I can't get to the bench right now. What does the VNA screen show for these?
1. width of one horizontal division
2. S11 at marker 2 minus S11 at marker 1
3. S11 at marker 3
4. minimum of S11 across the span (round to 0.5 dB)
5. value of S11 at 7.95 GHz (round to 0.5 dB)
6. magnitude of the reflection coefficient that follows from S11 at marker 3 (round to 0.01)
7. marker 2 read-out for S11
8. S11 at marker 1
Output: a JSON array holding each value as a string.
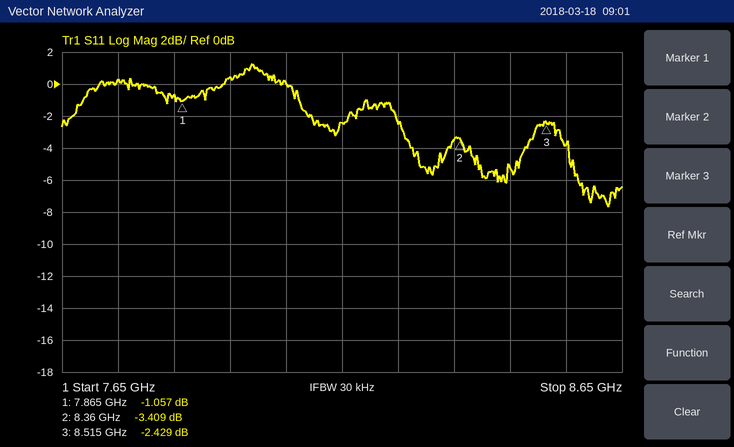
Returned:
["100 MHz", "-2.352 dB", "-2.429 dB", "-7.5 dB", "0.5 dB", "0.76", "-3.409 dB", "-1.057 dB"]
